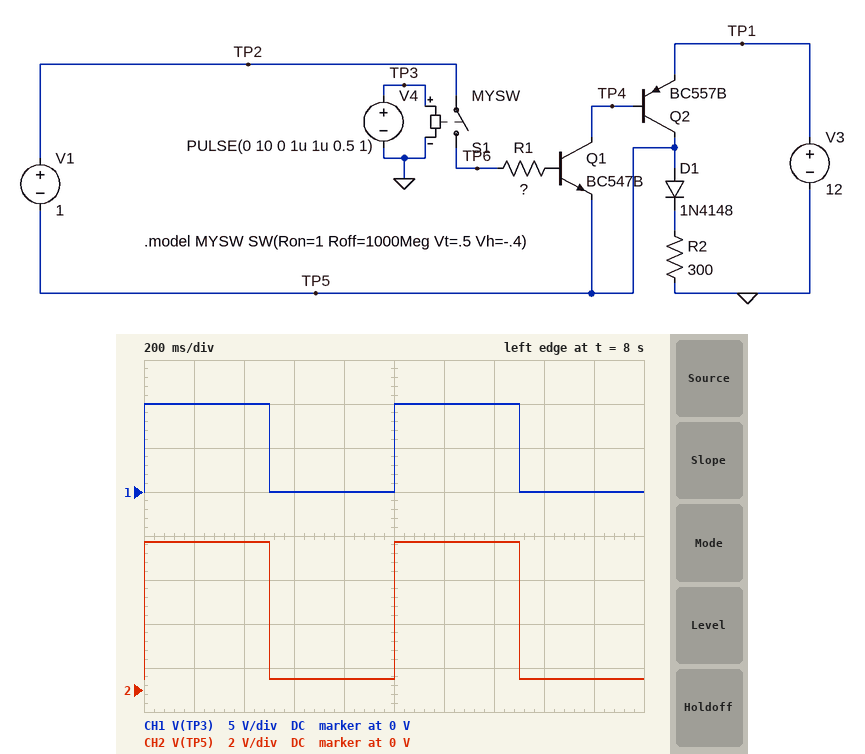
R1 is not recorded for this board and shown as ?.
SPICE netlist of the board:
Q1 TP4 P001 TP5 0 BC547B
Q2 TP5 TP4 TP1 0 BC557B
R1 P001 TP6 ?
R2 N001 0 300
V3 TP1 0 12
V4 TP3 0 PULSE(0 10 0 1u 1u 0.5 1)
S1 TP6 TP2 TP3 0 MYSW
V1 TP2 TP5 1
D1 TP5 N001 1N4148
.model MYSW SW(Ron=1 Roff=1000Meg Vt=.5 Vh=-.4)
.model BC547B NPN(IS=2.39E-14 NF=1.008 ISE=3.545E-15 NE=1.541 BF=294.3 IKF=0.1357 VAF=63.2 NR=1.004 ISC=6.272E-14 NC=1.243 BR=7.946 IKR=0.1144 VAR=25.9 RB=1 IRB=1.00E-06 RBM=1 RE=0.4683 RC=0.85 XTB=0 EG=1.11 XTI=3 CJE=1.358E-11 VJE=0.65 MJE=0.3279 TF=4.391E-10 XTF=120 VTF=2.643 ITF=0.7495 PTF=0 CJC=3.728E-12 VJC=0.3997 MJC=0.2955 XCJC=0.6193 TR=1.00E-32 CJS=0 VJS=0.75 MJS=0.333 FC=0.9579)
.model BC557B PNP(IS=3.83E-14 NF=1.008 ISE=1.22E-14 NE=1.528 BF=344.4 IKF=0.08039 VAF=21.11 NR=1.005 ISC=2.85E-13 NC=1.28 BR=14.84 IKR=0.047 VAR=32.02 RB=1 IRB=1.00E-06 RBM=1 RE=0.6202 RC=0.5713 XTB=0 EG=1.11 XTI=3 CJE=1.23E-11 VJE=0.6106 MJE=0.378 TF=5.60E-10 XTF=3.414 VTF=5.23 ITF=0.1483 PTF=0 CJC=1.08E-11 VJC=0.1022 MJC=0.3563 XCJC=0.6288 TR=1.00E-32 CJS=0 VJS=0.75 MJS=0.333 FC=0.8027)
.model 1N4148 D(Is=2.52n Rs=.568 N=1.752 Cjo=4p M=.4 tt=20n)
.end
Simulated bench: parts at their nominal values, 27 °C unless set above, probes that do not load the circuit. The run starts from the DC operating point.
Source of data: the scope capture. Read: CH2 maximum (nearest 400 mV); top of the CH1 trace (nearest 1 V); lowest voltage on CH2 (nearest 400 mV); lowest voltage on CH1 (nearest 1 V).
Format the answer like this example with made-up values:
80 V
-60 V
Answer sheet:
6.8 V
10 V
400 mV
0 V
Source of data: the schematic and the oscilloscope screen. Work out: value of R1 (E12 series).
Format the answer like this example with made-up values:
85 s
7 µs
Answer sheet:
2.2 MΩ
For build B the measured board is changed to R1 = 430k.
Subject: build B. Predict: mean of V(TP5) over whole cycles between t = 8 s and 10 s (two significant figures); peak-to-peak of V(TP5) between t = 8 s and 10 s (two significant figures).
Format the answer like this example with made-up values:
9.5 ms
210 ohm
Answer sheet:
5.8 V
11 V
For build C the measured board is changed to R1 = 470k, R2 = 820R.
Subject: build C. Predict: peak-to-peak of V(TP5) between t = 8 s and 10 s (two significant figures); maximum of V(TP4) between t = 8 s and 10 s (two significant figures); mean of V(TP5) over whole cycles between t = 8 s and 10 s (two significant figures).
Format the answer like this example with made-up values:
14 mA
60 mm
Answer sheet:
11 V
11 V
5.9 V
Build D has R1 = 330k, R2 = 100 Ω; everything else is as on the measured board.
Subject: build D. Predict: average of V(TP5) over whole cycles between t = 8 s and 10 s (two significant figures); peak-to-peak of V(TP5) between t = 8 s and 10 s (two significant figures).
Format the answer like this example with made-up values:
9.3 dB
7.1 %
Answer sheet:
4.3 V
7.7 V
